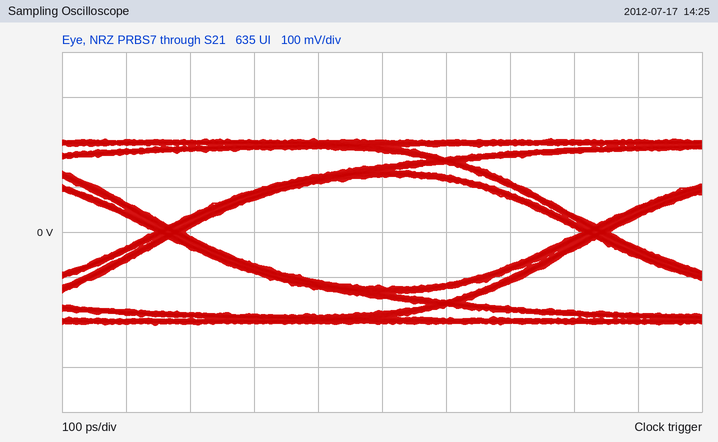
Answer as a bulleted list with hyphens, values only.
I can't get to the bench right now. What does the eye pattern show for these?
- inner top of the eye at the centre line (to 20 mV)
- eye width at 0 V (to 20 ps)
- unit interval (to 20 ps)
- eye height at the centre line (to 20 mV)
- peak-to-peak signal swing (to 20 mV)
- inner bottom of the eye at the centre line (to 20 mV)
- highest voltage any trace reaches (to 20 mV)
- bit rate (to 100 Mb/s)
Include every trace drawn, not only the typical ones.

- 120 mV
- 620 ps
- 660 ps
- 240 mV
- 420 mV
- -120 mV
- 200 mV
- 1.5 Gb/s
